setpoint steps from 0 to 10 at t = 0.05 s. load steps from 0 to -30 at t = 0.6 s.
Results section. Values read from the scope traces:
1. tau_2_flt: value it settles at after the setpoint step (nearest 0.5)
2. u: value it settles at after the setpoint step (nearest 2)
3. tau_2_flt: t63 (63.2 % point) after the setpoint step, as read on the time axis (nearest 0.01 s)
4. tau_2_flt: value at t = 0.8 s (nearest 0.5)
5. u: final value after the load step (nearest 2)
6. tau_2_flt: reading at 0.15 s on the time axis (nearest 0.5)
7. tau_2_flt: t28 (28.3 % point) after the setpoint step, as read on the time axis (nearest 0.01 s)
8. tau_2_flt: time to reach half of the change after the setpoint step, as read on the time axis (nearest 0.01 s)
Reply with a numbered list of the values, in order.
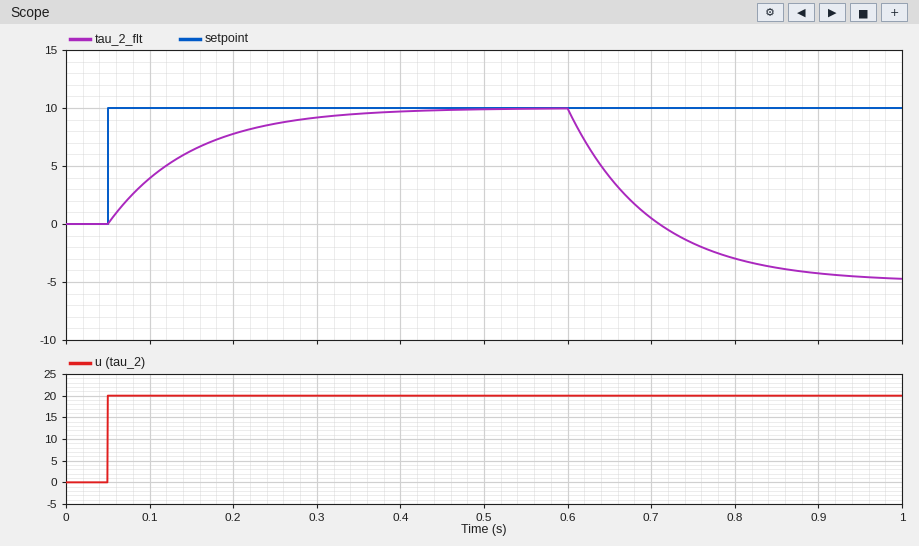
1. 10.0
2. 20
3. 0.15 s
4. -3.0
5. 20
6. 6.5
7. 0.08 s
8. 0.12 s
